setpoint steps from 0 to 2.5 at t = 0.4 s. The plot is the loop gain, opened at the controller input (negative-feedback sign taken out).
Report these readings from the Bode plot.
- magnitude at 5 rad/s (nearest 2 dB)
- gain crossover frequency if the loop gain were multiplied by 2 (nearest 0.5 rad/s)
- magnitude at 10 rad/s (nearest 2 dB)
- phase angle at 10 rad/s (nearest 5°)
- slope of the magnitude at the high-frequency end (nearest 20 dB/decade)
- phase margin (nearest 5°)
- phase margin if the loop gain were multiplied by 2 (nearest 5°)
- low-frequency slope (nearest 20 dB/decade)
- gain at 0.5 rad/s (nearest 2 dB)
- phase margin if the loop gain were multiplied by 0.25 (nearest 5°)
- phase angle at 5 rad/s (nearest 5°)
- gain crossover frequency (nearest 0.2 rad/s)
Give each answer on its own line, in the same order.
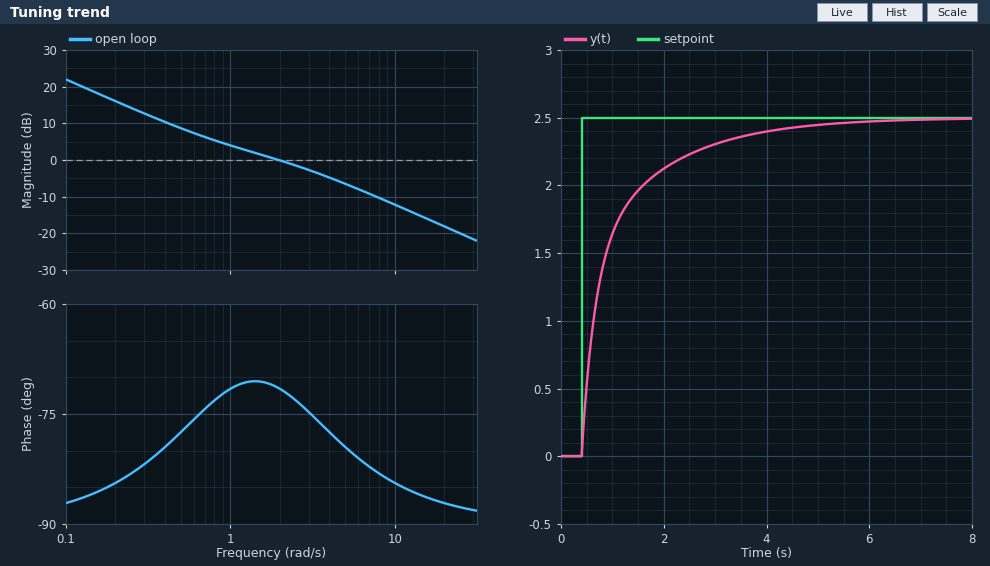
-6 dB
4.5 rad/s
-12 dB
-85°
-20 dB/decade
110°
100°
-20 dB/decade
8 dB
100°
-80°
2.0 rad/s
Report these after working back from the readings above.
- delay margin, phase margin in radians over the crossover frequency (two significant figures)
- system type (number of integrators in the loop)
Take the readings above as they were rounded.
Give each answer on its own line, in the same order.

0.96 s
1
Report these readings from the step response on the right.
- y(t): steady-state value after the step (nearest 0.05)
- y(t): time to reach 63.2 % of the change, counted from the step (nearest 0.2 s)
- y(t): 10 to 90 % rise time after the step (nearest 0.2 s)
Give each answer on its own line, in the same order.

2.50
0.6 s
2.2 s
